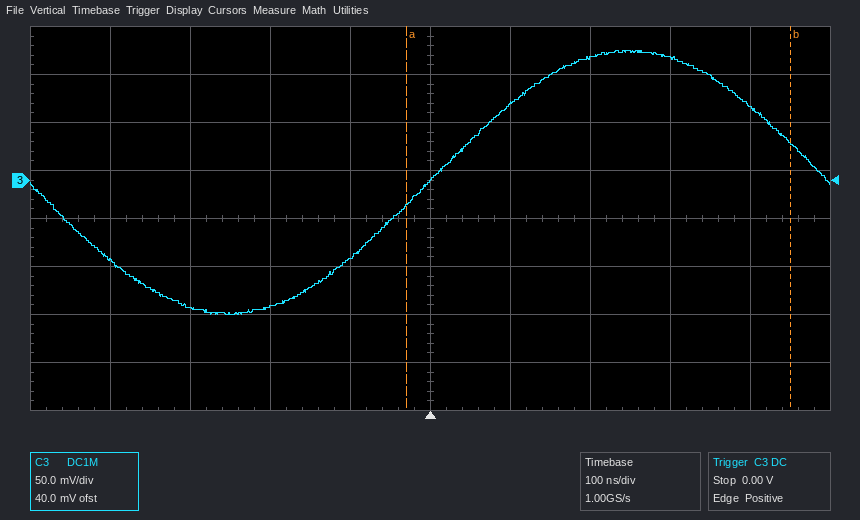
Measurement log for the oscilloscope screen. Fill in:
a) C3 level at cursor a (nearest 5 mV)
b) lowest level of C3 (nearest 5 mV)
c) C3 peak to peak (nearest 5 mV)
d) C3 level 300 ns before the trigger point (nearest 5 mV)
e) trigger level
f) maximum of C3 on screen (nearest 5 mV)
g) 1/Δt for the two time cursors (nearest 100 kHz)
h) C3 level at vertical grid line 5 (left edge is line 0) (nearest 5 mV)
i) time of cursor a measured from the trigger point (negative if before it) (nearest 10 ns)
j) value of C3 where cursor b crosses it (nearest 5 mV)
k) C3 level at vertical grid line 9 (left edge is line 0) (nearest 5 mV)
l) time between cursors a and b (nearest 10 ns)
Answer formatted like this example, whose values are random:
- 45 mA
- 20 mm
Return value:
- -25 mV
- -140 mV
- 275 mV
- -135 mV
- 0.00 V
- 135 mV
- 2.1 MHz
- 0 mV
- -30 ns
- 40 mV
- 75 mV
- 480 ns
